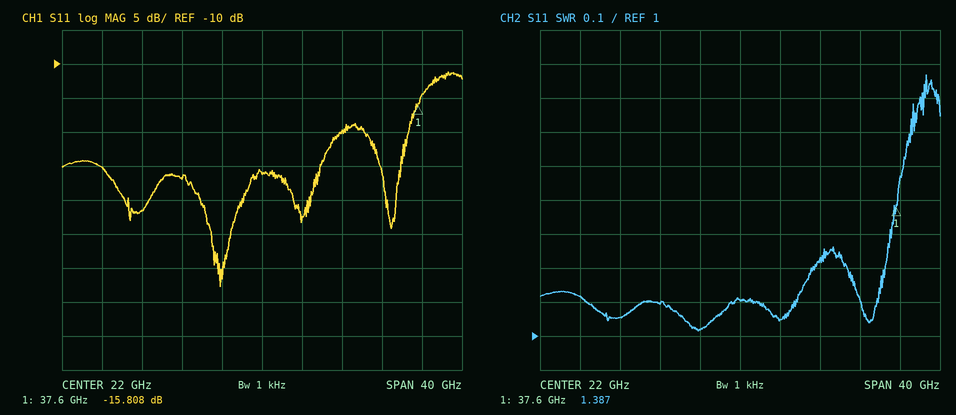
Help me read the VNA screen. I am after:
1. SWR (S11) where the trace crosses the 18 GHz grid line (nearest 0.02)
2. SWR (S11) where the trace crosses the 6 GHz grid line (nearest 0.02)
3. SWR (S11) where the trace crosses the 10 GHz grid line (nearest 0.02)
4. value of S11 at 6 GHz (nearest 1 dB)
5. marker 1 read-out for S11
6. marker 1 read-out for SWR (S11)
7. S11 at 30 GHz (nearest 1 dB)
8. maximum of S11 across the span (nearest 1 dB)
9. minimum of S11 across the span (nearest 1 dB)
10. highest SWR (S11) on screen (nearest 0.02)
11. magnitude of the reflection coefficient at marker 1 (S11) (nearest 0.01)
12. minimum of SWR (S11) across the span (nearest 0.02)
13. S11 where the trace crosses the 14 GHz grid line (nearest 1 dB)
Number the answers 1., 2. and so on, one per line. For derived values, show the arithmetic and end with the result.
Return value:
1. 1.02
2. 1.12
3. 1.06
4. -25 dB
5. -15.808 dB
6. 1.387
7. -20 dB
8. -11 dB
9. -43 dB
10. 1.76
11. 10^(-15.808/20) ≈ 0.16
12. 1.02
13. -27 dB
